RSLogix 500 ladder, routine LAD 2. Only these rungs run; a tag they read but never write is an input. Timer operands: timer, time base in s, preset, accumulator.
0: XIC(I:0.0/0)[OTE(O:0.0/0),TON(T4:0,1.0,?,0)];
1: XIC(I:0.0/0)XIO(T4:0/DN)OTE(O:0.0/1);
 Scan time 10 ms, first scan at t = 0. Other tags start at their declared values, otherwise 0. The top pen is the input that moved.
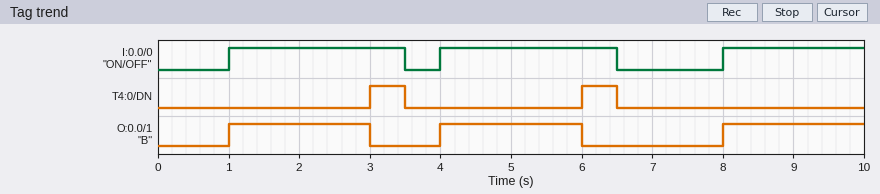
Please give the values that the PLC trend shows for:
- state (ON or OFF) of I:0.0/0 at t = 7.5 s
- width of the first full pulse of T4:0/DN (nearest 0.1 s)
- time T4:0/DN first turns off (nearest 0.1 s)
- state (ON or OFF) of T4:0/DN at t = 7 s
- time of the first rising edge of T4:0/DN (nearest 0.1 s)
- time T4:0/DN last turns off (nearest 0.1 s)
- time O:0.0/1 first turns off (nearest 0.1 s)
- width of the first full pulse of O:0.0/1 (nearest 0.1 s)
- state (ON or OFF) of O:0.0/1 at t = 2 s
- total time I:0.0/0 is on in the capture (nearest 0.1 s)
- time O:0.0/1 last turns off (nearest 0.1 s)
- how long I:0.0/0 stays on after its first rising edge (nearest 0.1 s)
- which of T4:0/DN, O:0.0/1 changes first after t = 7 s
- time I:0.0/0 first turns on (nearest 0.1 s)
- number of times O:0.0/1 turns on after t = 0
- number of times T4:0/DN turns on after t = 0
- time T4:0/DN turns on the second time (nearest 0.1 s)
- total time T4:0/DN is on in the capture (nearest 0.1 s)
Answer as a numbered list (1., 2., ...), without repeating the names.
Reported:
1. OFF
2. 0.5 s
3. 3.5 s
4. OFF
5. 3.0 s
6. 6.5 s
7. 3.0 s
8. 2.0 s
9. ON
10. 7.0 s
11. 6.0 s
12. 2.5 s
13. O:0.0/1
14. 1.0 s
15. 3
16. 2
17. 6.0 s
18. 1.0 s
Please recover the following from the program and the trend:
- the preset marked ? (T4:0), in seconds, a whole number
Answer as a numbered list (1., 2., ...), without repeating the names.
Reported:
1. 2 s
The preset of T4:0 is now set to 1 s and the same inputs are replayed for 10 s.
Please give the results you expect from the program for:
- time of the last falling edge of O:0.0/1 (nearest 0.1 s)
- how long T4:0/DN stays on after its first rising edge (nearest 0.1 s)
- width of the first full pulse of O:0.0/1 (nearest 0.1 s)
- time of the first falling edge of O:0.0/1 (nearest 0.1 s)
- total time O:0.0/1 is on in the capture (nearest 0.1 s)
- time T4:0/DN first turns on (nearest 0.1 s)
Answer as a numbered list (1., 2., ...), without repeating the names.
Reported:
1. 9.0 s
2. 1.5 s
3. 1.0 s
4. 2.0 s
5. 3.0 s
6. 2.0 s
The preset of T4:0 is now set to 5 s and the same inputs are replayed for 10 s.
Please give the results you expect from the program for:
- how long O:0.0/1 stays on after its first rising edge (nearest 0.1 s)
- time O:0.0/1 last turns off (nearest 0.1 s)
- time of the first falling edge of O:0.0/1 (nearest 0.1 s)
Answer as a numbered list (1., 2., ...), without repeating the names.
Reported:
1. 2.5 s
2. 6.5 s
3. 3.5 s
